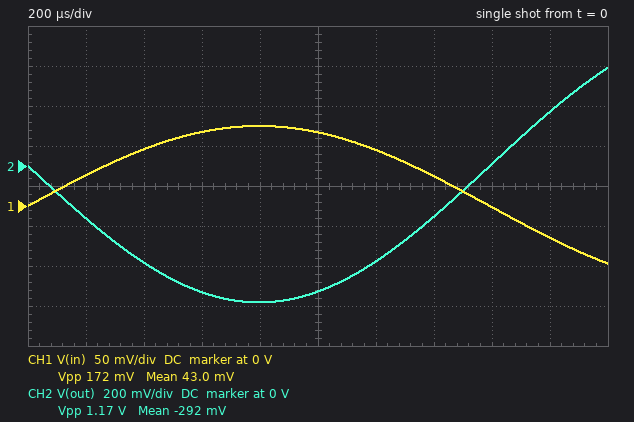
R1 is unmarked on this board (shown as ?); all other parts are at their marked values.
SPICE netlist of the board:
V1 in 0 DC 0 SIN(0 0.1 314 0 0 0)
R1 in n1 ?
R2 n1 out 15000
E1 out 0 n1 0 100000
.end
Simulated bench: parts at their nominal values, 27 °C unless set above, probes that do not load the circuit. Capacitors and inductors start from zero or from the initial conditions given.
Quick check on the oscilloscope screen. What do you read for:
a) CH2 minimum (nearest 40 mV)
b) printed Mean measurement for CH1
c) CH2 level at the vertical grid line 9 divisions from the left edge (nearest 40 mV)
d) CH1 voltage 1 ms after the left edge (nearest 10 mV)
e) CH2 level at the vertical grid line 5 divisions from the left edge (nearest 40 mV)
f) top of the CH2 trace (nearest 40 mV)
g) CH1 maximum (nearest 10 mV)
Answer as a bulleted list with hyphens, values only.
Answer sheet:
- -680 mV
- 43.0 mV
- 280 mV
- 90 mV
- -640 mV
- 480 mV
- 100 mV
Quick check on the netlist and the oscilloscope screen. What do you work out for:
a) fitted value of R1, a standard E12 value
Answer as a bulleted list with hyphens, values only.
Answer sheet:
- 2.2 kΩ
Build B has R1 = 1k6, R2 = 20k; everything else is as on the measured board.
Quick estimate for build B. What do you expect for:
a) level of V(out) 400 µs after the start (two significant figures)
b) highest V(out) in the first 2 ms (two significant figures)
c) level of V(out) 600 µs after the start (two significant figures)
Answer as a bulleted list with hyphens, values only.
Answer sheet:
- -890 mV
- 900 mV
- -1.2 V
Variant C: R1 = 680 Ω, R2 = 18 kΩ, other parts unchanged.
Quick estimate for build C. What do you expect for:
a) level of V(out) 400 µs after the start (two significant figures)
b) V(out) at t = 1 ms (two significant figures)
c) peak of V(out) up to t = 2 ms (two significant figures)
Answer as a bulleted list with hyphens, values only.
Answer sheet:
- -1.9 V
- -2.4 V
- 1.9 V
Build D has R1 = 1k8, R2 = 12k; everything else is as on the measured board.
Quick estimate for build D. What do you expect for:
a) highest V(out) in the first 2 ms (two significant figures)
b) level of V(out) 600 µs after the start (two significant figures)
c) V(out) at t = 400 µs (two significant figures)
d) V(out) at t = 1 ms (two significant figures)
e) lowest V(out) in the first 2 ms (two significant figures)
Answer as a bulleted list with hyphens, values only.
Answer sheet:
- 480 mV
- -620 mV
- -470 mV
- -610 mV
- -670 mV
